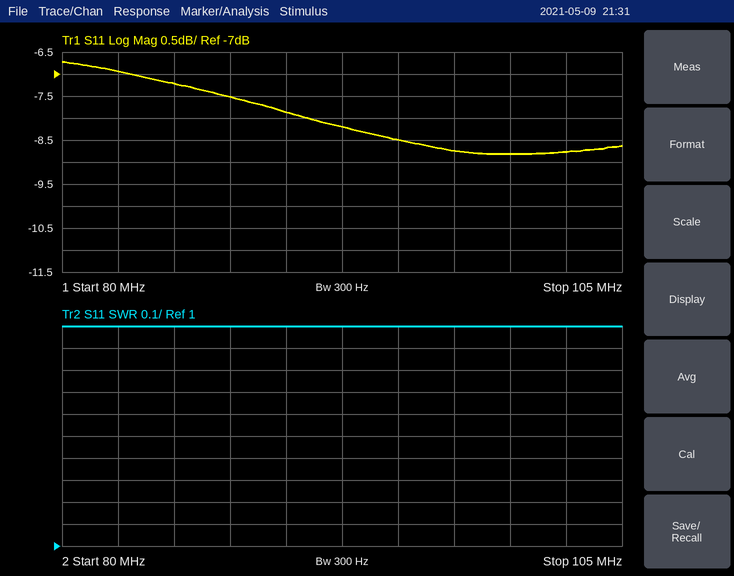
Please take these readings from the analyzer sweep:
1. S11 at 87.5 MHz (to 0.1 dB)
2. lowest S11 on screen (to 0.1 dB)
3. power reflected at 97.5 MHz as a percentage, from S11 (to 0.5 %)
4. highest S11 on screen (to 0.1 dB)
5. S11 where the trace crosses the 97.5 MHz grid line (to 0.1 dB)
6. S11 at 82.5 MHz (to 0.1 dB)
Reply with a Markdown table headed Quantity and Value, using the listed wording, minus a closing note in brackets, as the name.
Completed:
| Quantity | Value |
|---|---|
| S11 at 87.5 MHz | -7.5 dB |
| lowest S11 on screen | -8.8 dB |
| power reflected at 97.5 MHz as a percentage, from S11 | 13.5 % |
| highest S11 on screen | -6.7 dB |
| S11 where the trace crosses the 97.5 MHz grid line | -8.7 dB |
| S11 at 82.5 MHz | -6.9 dB |
